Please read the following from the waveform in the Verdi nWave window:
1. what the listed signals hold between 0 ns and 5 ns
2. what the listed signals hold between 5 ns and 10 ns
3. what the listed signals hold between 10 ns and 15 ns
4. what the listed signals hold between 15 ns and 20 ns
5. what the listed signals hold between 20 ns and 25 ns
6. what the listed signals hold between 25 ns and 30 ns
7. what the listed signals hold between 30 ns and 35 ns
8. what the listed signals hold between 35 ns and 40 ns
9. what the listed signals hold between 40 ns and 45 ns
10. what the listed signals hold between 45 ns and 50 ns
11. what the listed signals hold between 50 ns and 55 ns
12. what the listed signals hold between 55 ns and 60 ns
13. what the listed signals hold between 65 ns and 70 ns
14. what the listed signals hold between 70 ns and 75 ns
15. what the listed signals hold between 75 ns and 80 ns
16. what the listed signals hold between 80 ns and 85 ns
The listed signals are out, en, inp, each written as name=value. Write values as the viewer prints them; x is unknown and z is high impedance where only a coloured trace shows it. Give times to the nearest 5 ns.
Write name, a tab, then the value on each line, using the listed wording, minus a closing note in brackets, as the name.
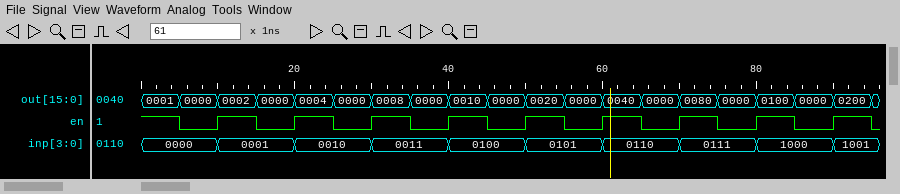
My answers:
what the listed signals hold between 0 ns and 5 ns	out=0001, en=1, inp=0000
what the listed signals hold between 5 ns and 10 ns	out=0000, en=0, inp=0000
what the listed signals hold between 10 ns and 15 ns	out=0002, en=1, inp=0001
what the listed signals hold between 15 ns and 20 ns	out=0000, en=0, inp=0001
what the listed signals hold between 20 ns and 25 ns	out=0004, en=1, inp=0010
what the listed signals hold between 25 ns and 30 ns	out=0000, en=0, inp=0010
what the listed signals hold between 30 ns and 35 ns	out=0008, en=1, inp=0011
what the listed signals hold between 35 ns and 40 ns	out=0000, en=0, inp=0011
what the listed signals hold between 40 ns and 45 ns	out=0010, en=1, inp=0100
what the listed signals hold between 45 ns and 50 ns	out=0000, en=0, inp=0100
what the listed signals hold between 50 ns and 55 ns	out=0020, en=1, inp=0101
what the listed signals hold between 55 ns and 60 ns	out=0000, en=0, inp=0101
what the listed signals hold between 65 ns and 70 ns	out=0000, en=0, inp=0110
what the listed signals hold between 70 ns and 75 ns	out=0080, en=1, inp=0111
what the listed signals hold between 75 ns and 80 ns	out=0000, en=0, inp=0111
what the listed signals hold between 80 ns and 85 ns	out=0100, en=1, inp=1000
